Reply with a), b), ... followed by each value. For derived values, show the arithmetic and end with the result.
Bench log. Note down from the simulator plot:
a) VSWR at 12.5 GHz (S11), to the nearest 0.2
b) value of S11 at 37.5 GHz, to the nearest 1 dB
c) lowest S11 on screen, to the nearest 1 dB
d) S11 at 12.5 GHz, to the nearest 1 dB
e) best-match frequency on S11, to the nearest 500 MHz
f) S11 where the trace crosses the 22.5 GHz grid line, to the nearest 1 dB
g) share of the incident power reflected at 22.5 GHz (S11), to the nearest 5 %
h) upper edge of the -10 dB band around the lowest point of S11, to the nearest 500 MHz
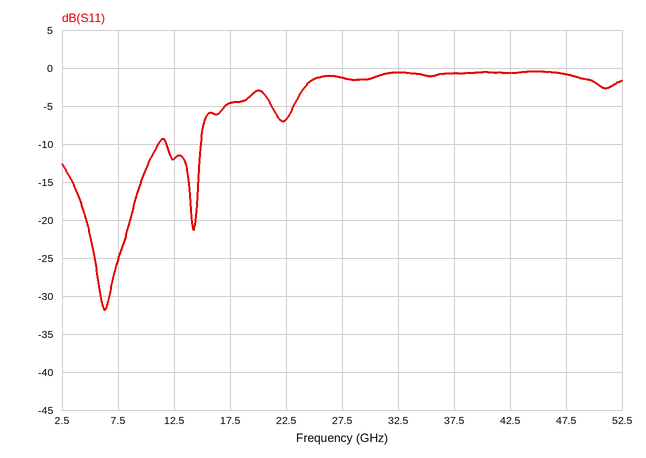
a) |Γ| = 10^(-12/20) = 0.2512; VSWR = (1 + 0.2512)/(1 − 0.2512) ≈ 1.67, so 1.6 to the nearest 0.2
b) -1 dB
c) -32 dB
d) -12 dB
e) 6.5 GHz
f) -7 dB
g) 10^(-7/10) ≈ 20 %
h) 11.0 GHz
